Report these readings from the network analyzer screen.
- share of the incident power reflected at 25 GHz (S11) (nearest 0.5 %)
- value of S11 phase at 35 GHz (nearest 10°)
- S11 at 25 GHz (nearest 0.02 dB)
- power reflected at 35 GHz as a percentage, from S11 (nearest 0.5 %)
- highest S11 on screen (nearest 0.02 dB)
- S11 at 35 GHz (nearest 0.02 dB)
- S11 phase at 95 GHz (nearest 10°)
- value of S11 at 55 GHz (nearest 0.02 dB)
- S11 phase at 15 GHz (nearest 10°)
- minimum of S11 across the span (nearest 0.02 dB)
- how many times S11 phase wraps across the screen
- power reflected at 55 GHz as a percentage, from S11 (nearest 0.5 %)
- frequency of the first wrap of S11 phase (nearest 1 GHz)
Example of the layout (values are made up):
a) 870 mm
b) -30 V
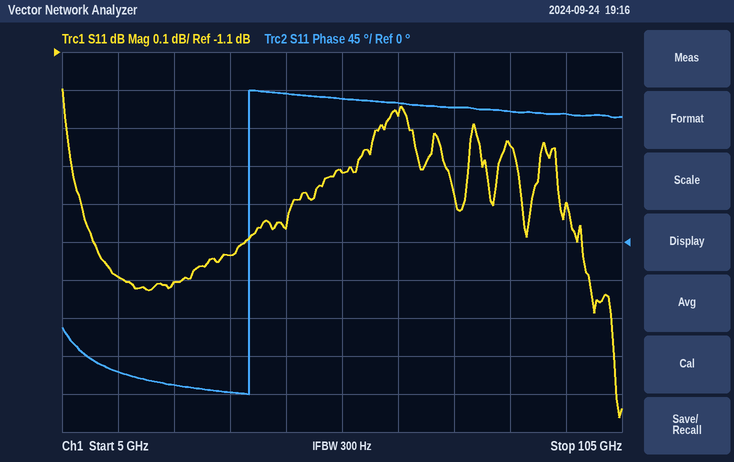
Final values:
a) 67.5 %
b) -180°
c) -1.70 dB
d) 68.5 %
e) -1.20 dB
f) -1.64 dB
g) 150°
h) -1.42 dB
i) -150°
j) -2.06 dB
k) 1
l) 72.0 %
m) 38 GHz
